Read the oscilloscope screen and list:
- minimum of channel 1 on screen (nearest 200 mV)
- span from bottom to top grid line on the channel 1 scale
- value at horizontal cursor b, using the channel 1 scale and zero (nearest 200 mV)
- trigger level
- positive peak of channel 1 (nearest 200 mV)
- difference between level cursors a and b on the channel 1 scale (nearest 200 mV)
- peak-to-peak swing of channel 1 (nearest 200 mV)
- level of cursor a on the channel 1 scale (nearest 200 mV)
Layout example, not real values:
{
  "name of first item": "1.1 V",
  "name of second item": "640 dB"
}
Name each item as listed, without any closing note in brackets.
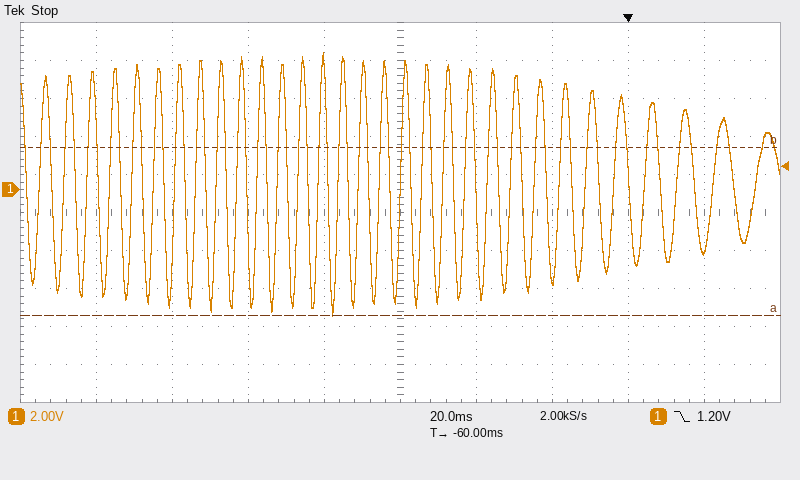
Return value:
{
  "minimum of channel 1 on screen": "-6.6 V",
  "span from bottom to top grid line on the channel 1 scale": "20 V",
  "value at horizontal cursor b, using the channel 1 scale and zero": "2.2 V",
  "trigger level": "1.20 V",
  "positive peak of channel 1": "7.2 V",
  "difference between level cursors a and b on the channel 1 scale": "8.8 V",
  "peak-to-peak swing of channel 1": "13.8 V",
  "level of cursor a on the channel 1 scale": "-6.6 V"
}
